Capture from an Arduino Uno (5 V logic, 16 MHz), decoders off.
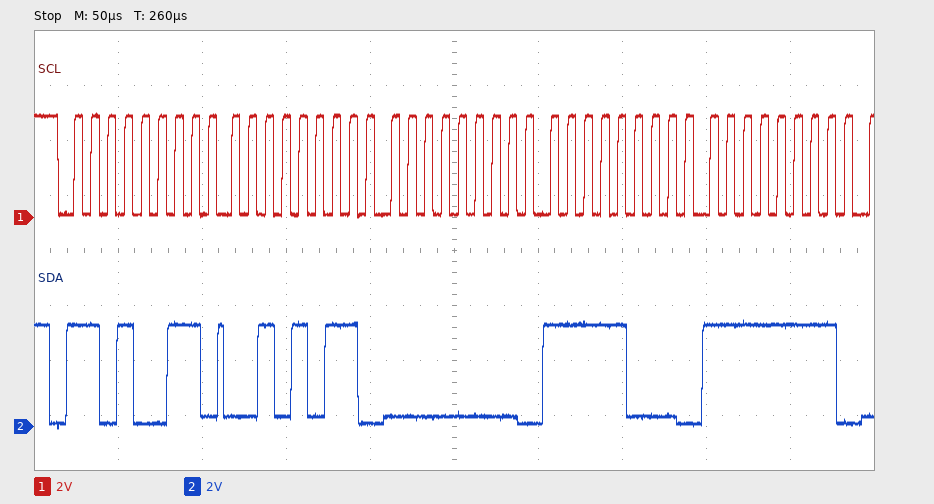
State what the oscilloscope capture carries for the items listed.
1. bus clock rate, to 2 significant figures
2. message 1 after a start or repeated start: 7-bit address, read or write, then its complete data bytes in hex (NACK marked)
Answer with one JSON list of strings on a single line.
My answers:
["100 kHz", "0x69 read: 2B 00 F8 FF"]
